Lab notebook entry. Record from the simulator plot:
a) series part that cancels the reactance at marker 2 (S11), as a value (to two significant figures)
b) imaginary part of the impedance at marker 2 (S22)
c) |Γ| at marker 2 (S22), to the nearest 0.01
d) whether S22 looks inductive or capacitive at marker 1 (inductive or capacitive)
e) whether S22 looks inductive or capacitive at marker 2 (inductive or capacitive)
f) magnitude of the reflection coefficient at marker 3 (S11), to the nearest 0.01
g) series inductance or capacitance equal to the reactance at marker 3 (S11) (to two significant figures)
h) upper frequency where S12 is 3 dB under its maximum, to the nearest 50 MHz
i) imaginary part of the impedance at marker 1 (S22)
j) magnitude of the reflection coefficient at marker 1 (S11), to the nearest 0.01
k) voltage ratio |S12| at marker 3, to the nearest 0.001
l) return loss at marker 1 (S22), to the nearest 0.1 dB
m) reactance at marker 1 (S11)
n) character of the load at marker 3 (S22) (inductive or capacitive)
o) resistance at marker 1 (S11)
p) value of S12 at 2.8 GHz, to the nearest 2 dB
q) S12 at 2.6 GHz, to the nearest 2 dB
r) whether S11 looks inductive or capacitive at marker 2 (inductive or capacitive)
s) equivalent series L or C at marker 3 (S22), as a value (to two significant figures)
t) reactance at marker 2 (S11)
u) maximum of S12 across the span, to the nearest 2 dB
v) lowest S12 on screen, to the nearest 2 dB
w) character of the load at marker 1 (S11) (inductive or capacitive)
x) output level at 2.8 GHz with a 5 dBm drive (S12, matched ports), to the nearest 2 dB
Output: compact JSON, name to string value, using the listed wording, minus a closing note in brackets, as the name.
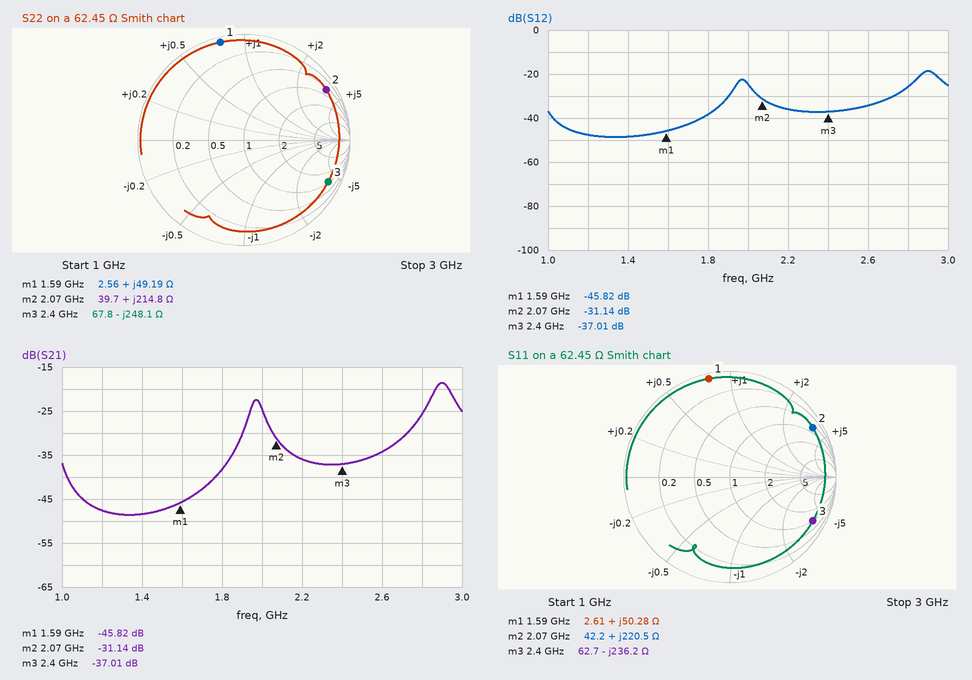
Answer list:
{"series part that cancels the reactance at marker 2 (S11), as a value": "350 fF", "imaginary part of the impedance at marker 2": "+214.8 Ω", "|Γ| at marker 2 (S22), to the nearest 0.01": "0.91", "whether S22 looks inductive or capacitive at marker 1": "inductive", "whether S22 looks inductive or capacitive at marker 2": "inductive", "magnitude of the reflection coefficient at marker 3 (S11), to the nearest 0.01": "0.88", "series inductance or capacitance equal to the reactance at marker 3 (S11)": "280 fF", "upper frequency where S12 is 3 dB under its maximum, to the nearest 50 MHz": "2.95 GHz", "imaginary part of the impedance at marker 1": "+49.19 Ω", "magnitude of the reflection coefficient at marker 1 (S11), to the nearest 0.01": "0.95", "voltage ratio |S12| at marker 3, to the nearest 0.001": "0.014", "return loss at marker 1 (S22), to the nearest 0.1 dB": "0.4 dB", "reactance at marker 1": "+50.28 Ω", "character of the load at marker 3 (S22)": "capacitive", "resistance at marker 1": "2.61 Ω", "value of S12 at 2.8 GHz, to the nearest 2 dB": "-26 dB", "S12 at 2.6 GHz, to the nearest 2 dB": "-34 dB", "whether S11 looks inductive or capacitive at marker 2": "inductive", "equivalent series L or C at marker 3 (S22), as a value": "270 fF", "reactance at marker 2": "+220.5 Ω", "maximum of S12 across the span, to the nearest 2 dB": "-18 dB", "lowest S12 on screen, to the nearest 2 dB": "-48 dB", "character of the load at marker 1 (S11)": "inductive", "output level at 2.8 GHz with a 5 dBm drive (S12, matched ports), to the nearest 2 dB": "-20 dBm"}
